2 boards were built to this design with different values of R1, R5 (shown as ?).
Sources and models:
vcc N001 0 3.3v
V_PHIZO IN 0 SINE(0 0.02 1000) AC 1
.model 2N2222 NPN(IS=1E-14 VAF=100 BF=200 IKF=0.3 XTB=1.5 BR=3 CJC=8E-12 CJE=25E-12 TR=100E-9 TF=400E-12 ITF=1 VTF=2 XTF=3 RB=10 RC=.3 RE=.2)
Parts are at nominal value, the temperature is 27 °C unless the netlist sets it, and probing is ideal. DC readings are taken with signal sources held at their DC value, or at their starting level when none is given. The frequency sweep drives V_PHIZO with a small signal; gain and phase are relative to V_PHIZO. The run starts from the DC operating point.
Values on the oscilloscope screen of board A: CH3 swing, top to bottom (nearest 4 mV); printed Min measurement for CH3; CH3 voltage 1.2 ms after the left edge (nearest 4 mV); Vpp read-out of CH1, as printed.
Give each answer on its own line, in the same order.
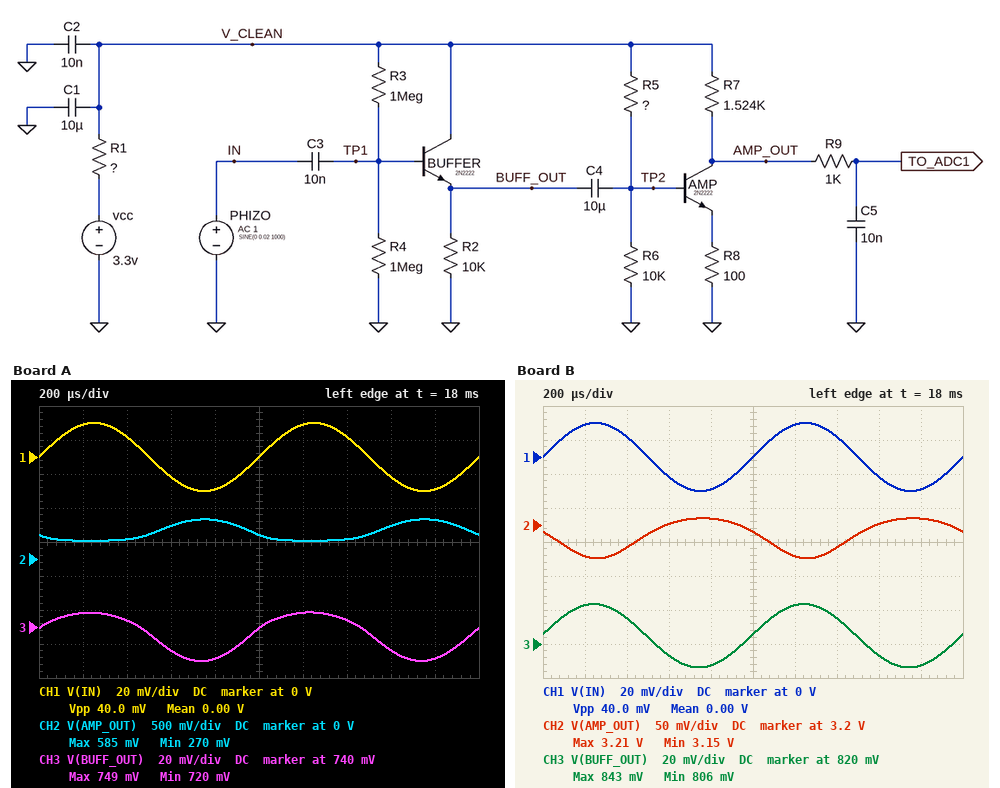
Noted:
28 mV
720 mV
748 mV
40.0 mV
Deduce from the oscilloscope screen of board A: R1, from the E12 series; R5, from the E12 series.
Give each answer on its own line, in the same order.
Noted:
150 Ω
22 kΩ
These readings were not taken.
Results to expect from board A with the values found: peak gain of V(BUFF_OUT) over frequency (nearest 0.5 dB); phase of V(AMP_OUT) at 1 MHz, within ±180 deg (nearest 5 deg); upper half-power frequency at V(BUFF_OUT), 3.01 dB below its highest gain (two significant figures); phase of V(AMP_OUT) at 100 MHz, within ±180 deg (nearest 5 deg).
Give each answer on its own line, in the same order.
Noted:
-1.0 dB
145 deg
3.3 GHz
30 deg
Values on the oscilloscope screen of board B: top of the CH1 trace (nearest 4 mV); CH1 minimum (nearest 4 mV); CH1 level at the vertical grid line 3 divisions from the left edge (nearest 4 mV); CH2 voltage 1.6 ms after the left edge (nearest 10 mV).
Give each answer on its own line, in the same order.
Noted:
20 mV
-20 mV
-12 mV
3.20 V
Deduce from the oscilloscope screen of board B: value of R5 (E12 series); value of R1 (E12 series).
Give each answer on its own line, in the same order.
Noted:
47 kΩ
390 Ω
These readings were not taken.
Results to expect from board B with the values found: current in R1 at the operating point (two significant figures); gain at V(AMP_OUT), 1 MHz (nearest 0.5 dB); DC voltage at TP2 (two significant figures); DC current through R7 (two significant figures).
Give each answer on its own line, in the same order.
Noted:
170 µA
-5.0 dB
570 mV
29 µA
